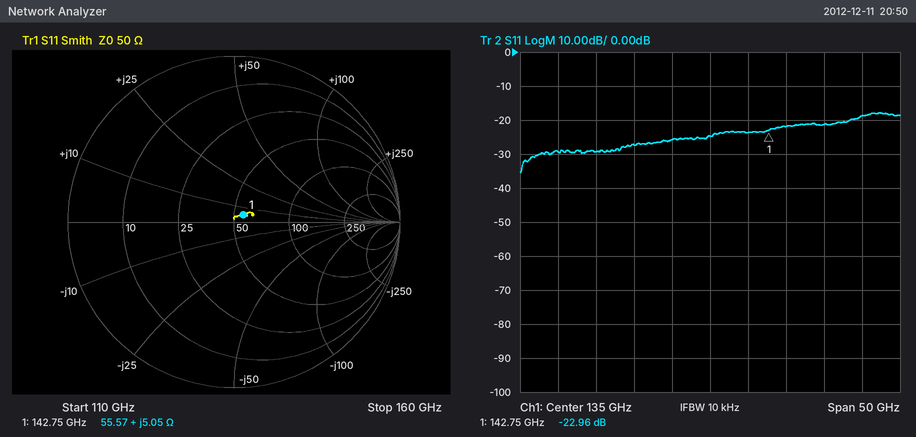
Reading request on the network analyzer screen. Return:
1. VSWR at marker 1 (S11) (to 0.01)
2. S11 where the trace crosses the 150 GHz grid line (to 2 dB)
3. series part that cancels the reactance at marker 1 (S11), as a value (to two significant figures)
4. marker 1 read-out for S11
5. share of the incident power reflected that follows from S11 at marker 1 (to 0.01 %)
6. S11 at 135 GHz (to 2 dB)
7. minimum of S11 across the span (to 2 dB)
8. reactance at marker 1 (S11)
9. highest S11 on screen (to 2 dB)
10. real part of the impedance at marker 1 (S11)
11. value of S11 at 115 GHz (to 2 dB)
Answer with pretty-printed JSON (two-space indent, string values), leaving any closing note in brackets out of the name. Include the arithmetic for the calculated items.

{
  "VSWR at marker 1 (S11)": "1.15",
  "S11 where the trace crosses the 150 GHz grid line": "-22 dB",
  "series part that cancels the reactance at marker 1 (S11), as a value": "C = 1/(2π × 142.75 GHz × 5.05 Ω) ≈ 221 fF, so 220 fF to two significant figures",
  "marker 1 read-out for S11": "-22.96 dB",
  "share of the incident power reflected that follows from S11 at marker 1": "10^(-22.96/10) ≈ 0.51 %",
  "S11 at 135 GHz": "-24 dB",
  "minimum of S11 across the span": "-36 dB",
  "reactance at marker 1": "+5.05 Ω",
  "highest S11 on screen": "-18 dB",
  "real part of the impedance at marker 1": "55.57 Ω",
  "value of S11 at 115 GHz": "-30 dB"
}
